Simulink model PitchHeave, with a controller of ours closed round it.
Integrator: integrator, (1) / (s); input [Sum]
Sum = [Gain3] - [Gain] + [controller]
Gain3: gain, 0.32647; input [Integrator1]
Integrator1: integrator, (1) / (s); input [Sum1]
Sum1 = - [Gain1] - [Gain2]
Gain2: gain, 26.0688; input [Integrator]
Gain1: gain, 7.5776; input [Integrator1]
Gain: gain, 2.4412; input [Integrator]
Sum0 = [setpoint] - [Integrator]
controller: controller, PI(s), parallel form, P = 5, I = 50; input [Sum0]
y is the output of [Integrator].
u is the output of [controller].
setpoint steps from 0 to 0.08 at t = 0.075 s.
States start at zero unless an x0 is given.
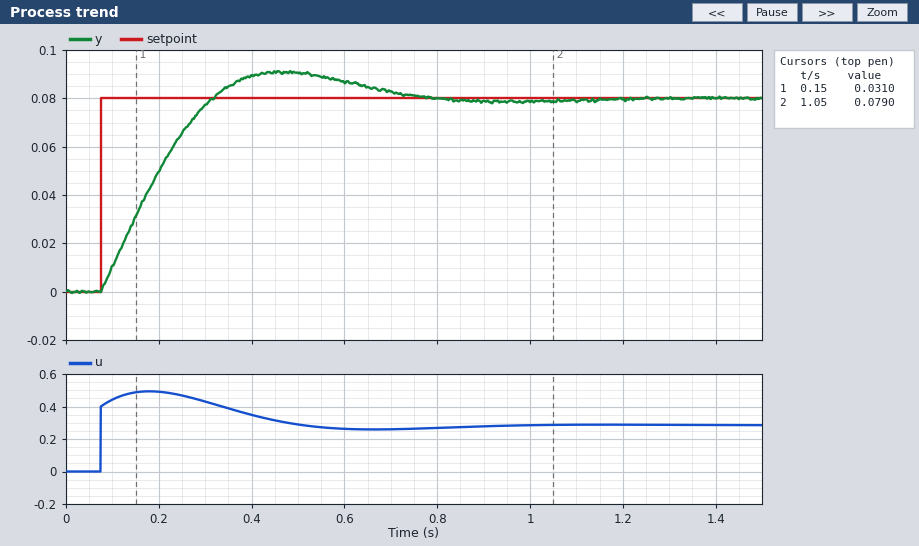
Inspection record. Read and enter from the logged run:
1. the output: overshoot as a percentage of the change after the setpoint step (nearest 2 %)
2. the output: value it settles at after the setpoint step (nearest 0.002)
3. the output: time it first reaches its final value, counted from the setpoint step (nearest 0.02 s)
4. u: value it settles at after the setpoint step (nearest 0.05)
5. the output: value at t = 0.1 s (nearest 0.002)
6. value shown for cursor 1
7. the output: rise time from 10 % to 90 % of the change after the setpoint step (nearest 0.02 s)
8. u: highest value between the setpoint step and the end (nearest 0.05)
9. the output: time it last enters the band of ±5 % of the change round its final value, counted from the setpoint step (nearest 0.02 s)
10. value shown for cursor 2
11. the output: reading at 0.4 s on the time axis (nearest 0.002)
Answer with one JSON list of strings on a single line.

["14 %", "0.080", "0.24 s", "0.30", "0.010", "0.0310", "0.18 s", "0.50", "0.60 s", "0.0790", "0.090"]
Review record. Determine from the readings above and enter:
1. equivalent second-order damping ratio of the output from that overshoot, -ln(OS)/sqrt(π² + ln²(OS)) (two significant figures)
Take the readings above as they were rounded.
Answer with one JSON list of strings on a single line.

["0.53"]
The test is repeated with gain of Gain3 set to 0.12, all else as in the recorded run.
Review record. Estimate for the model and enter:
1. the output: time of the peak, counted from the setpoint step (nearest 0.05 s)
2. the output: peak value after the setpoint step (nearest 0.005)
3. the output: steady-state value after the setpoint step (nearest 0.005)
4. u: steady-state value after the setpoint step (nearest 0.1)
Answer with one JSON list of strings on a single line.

["0.40 s", "0.095", "0.080", "0.2"]
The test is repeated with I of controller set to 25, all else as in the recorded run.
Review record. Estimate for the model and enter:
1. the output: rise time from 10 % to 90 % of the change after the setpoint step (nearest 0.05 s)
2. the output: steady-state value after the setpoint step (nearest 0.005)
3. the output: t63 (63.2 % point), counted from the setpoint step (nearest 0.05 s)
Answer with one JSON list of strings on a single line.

["0.30 s", "0.080", "0.15 s"]
